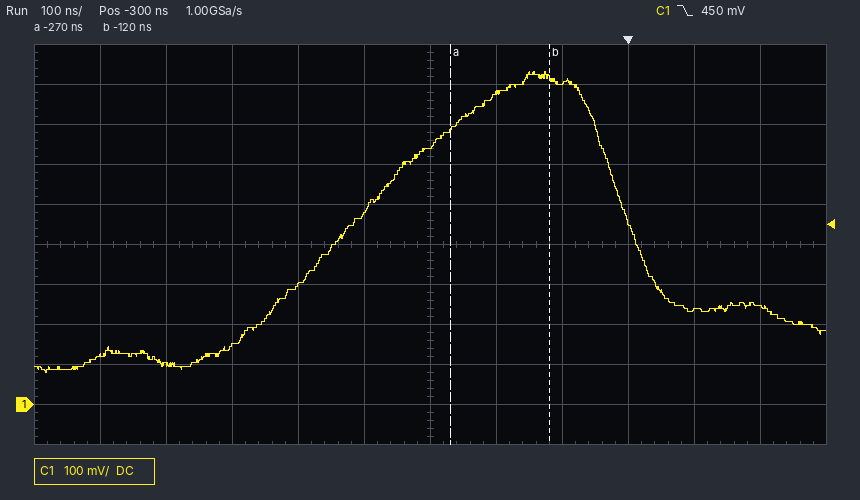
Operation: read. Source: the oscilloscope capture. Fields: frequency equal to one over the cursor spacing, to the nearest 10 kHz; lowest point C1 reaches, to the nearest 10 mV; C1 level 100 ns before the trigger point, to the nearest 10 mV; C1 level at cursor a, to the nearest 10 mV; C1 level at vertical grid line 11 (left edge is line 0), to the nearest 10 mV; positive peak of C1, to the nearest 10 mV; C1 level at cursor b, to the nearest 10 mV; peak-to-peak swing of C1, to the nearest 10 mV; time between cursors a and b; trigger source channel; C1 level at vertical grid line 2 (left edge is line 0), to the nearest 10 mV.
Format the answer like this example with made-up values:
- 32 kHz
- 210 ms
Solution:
- 6.67 MHz
- 80 mV
- 800 mV
- 690 mV
- 240 mV
- 830 mV
- 820 mV
- 750 mV
- 150 ns
- C1
- 100 mV
